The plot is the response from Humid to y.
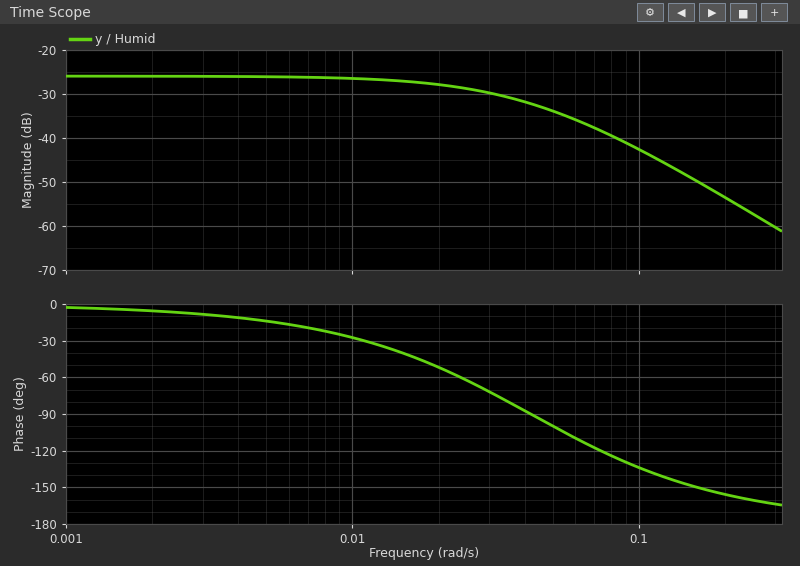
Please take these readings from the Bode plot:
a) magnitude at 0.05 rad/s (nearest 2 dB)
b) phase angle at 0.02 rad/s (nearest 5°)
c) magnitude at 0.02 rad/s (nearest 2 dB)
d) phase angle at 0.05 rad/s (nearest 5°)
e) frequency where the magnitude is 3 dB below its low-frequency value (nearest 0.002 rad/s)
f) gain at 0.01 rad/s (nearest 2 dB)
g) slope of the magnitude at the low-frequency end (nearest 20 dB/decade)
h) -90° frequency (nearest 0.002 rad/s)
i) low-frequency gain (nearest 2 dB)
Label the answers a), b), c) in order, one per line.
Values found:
a) -34 dB
b) -50°
c) -28 dB
d) -100°
e) 0.026 rad/s
f) -26 dB
g) 0 dB/decade
h) 0.042 rad/s
i) -26 dB
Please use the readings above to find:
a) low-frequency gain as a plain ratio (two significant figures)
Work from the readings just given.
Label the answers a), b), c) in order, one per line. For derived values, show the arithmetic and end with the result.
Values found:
a) 10^(-26 / 20) = 0.050
